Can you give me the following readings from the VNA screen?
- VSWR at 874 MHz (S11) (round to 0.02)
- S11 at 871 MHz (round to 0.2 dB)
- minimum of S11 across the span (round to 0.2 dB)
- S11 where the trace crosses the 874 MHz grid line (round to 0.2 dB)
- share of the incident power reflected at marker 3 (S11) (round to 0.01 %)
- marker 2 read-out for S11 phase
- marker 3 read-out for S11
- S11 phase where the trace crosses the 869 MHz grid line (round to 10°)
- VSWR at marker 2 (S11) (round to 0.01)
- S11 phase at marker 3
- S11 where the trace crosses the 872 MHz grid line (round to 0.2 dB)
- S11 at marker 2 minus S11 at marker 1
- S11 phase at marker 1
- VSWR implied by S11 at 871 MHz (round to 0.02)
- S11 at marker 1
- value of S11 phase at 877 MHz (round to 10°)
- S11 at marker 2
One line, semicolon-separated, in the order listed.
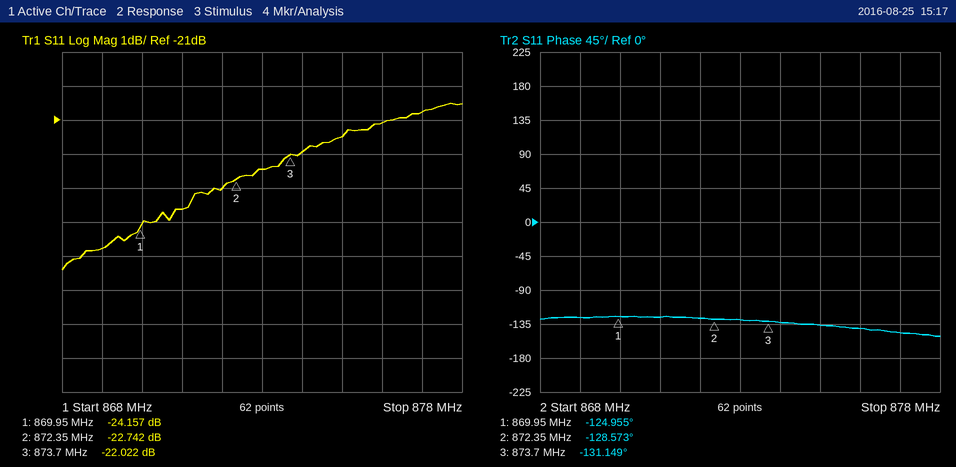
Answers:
1.18; -23.6 dB; -25.4 dB; -22.0 dB; 0.63 %; -128.573°; -22.022 dB; -130°; 1.16; -131.149°; -23.0 dB; 1.415 dB; -124.955°; 1.14; -24.157 dB; -150°; -22.742 dB
